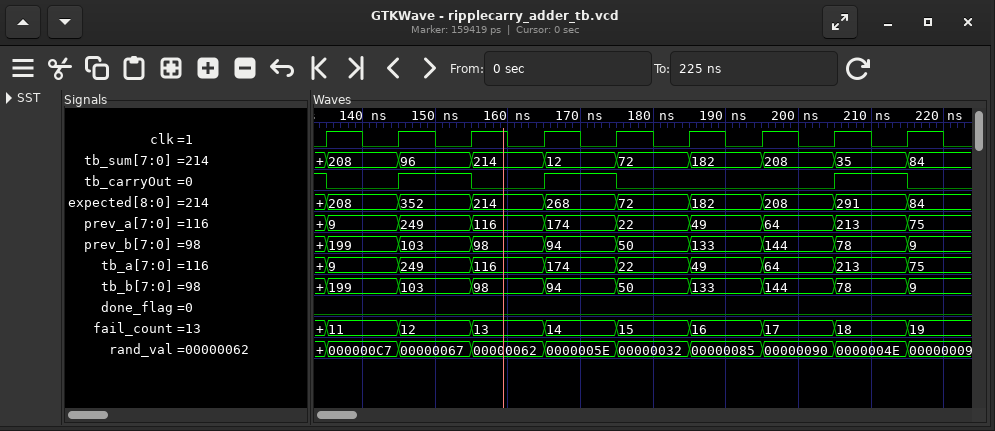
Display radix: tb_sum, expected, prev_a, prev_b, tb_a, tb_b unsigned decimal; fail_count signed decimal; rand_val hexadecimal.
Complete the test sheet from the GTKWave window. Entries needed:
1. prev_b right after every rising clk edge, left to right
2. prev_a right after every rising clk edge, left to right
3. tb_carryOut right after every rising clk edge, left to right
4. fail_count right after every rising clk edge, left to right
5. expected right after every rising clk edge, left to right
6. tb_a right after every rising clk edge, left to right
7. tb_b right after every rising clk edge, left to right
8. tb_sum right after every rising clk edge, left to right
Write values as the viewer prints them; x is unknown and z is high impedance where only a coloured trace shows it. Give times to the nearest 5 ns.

199, 103, 98, 94, 50, 133, 144, 78, 9
9, 249, 116, 174, 22, 49, 64, 213, 75
0 1 0 1 0 0 0 1 0
11, 12, 13, 14, 15, 16, 17, 18, 19
208, 352, 214, 268, 72, 182, 208, 291, 84
9, 249, 116, 174, 22, 49, 64, 213, 75
199, 103, 98, 94, 50, 133, 144, 78, 9
208, 96, 214, 12, 72, 182, 208, 35, 84
